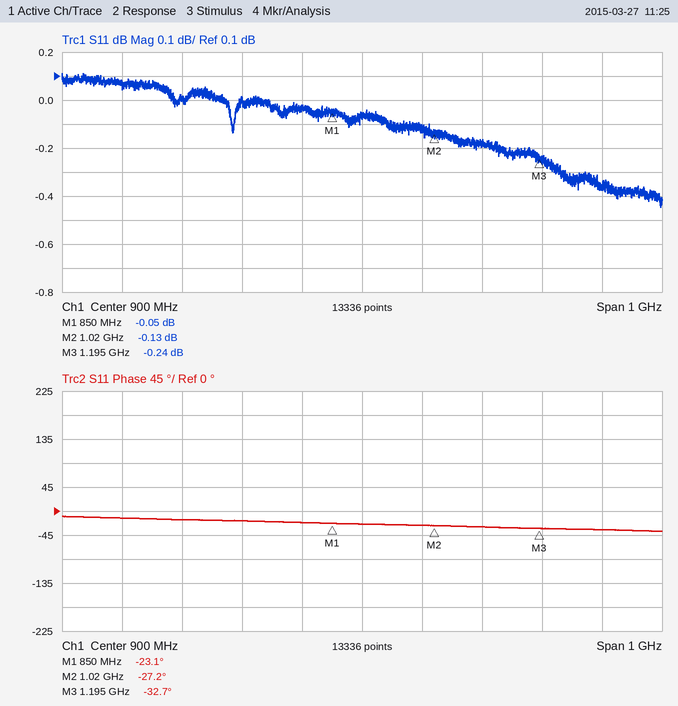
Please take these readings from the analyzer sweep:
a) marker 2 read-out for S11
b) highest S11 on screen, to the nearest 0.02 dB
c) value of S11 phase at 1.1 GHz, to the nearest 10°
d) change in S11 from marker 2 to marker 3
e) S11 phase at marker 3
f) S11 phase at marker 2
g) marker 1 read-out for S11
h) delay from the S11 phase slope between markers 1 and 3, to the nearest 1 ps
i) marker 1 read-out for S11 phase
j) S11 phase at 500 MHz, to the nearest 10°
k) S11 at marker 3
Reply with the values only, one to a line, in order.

-0.13 dB
0.12 dB
-30°
-0.11 dB
-32.7°
-27.2°
-0.05 dB
77 ps
-23.1°
-10°
-0.24 dB
